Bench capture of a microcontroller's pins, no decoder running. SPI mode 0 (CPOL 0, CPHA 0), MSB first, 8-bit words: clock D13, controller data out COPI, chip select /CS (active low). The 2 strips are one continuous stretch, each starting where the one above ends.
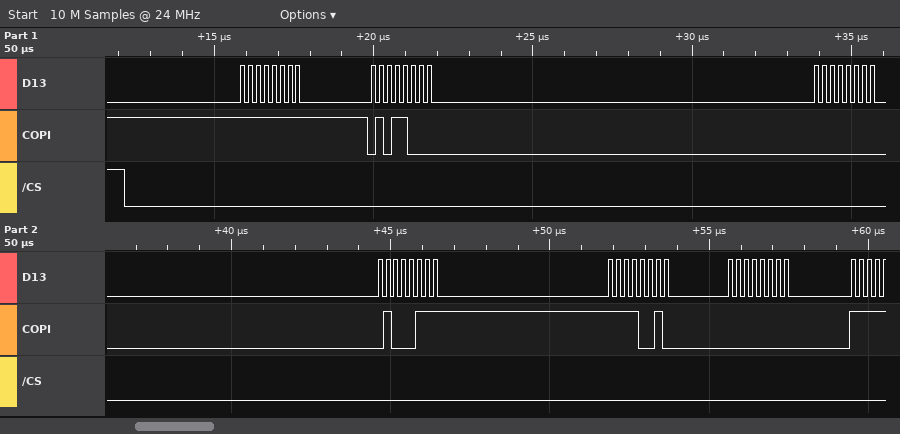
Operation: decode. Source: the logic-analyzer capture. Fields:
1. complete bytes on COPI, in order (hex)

FF 58 00 47 F2 00
